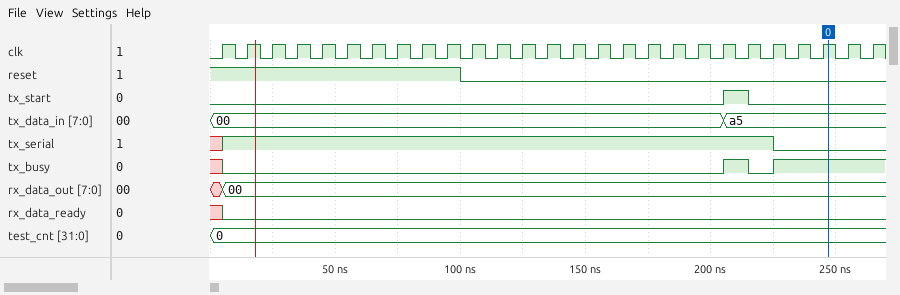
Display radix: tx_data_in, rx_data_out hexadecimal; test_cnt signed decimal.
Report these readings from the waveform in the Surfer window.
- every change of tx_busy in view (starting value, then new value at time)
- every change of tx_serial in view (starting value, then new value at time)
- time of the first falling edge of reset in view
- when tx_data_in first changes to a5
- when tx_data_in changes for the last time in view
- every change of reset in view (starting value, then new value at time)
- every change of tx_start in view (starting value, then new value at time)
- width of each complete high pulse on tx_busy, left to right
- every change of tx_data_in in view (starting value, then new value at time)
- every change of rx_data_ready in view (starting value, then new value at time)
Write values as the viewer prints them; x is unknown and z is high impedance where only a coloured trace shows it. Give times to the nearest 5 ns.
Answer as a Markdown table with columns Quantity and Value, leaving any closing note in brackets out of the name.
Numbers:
| Quantity | Value |
|---|---|
| every change of tx_busy in view | x, 0 at 5 ns, 1 at 205 ns, 0 at 215 ns, 1 at 225 ns |
| every change of tx_serial in view | x, 1 at 5 ns, 0 at 225 ns |
| time of the first falling edge of reset in view | 100 ns |
| when tx_data_in first changes to a5 | 205 ns |
| when tx_data_in changes for the last time in view | 205 ns |
| every change of reset in view | 1, 0 at 100 ns |
| every change of tx_start in view | 0, 1 at 205 ns, 0 at 215 ns |
| width of each complete high pulse on tx_busy, left to right | 10 ns |
| every change of tx_data_in in view | 00, a5 at 205 ns |
| every change of rx_data_ready in view | x, 0 at 5 ns |
